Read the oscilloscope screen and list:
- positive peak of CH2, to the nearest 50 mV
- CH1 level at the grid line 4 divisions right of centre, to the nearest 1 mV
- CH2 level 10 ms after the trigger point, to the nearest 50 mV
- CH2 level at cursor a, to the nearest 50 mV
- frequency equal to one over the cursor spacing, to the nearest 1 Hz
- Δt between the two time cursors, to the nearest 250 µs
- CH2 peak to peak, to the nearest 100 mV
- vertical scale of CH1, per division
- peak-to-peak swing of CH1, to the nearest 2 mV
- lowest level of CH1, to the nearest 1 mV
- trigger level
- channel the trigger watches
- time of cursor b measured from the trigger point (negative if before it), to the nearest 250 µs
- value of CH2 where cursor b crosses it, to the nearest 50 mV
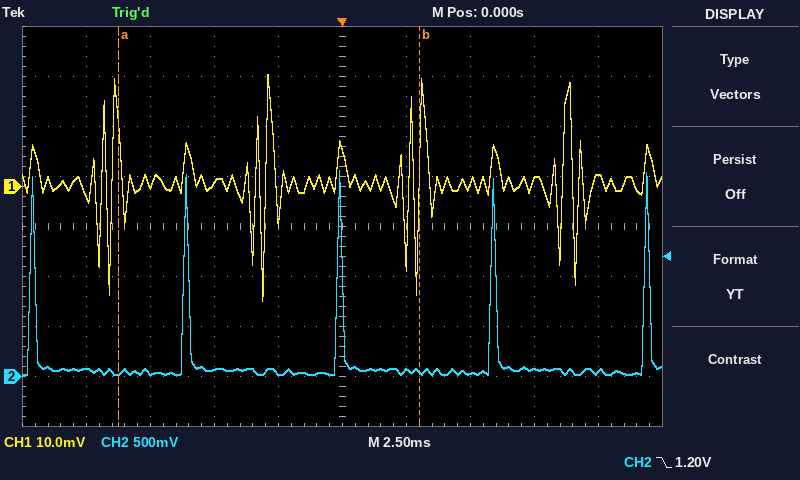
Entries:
2.05 V
2 mV
50 mV
50 mV
85 Hz
11.75 ms
2.00 V
10 mV
46 mV
-23 mV
1.20 V
CH2
+3.00 ms
50 mV
